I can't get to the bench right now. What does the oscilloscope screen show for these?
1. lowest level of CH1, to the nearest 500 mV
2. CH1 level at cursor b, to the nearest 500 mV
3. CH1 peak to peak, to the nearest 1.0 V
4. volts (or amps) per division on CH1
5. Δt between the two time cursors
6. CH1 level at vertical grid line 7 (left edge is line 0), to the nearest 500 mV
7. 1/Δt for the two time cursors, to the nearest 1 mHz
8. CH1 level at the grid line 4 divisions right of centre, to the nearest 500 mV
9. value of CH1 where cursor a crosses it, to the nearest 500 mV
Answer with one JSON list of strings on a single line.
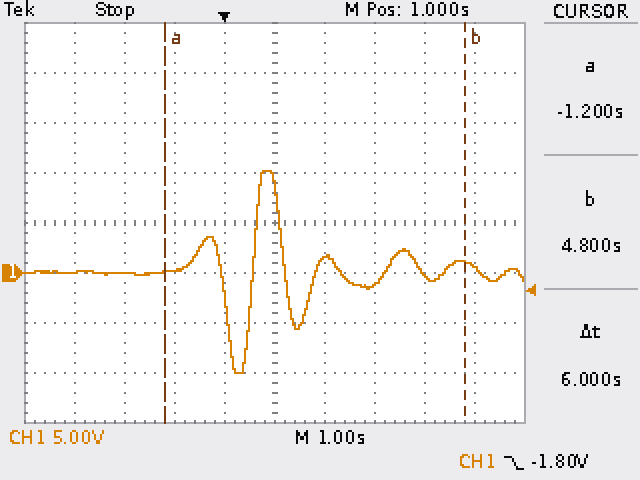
["-10.0 V", "1.0 V", "20.0 V", "5 V", "6 s", "-1.0 V", "167 mHz", "500 mV", "0.0 V"]
